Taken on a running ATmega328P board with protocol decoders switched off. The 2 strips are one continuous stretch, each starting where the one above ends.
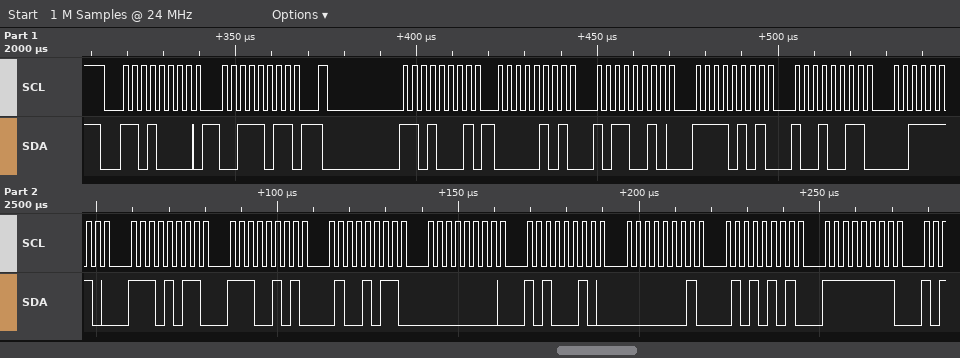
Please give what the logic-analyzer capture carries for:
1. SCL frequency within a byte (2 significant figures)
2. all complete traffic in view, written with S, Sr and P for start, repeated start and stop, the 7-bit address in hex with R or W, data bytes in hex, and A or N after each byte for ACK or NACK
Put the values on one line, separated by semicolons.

400 kHz; S 68W A 3B A Sr 68R A 05 A B2 A F5 A 93 A 3E A EB A E5 A 4B A 00 A A2 A 01 A 55 A FF A
